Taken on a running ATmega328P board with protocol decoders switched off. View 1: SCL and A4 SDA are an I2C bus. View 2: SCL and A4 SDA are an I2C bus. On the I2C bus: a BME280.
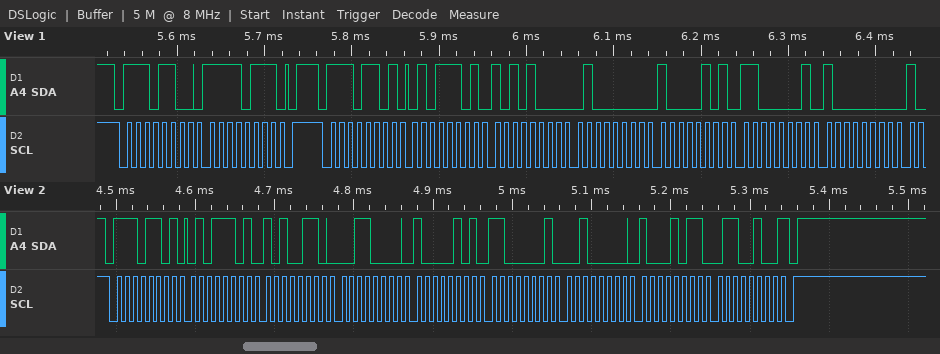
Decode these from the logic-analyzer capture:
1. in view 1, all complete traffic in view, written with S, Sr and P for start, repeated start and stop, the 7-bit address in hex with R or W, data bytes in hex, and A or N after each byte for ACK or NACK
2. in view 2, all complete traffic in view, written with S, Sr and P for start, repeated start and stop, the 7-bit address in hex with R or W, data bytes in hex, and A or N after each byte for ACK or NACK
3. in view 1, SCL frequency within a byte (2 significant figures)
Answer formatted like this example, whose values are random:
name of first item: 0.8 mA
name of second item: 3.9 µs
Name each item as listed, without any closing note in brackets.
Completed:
in view 1, all complete traffic in view, written with S, Sr and P for start, repeated start and stop, the 7-bit address in hex with R or W, data bytes in hex, and A or N after each byte for ACK or NACK: S 76W A F7 A P S 76R A 5D A A8 A 40 A 85 A C1 A 80 A
in view 2, all complete traffic in view, written with S, Sr and P for start, repeated start and stop, the 7-bit address in hex with R or W, data bytes in hex, and A or N after each byte for ACK or NACK: S 76R A 5D A A6 A 30 A 85 A C1 A 20 A 8B A 64 N P
in view 1, SCL frequency within a byte: 100 kHz
